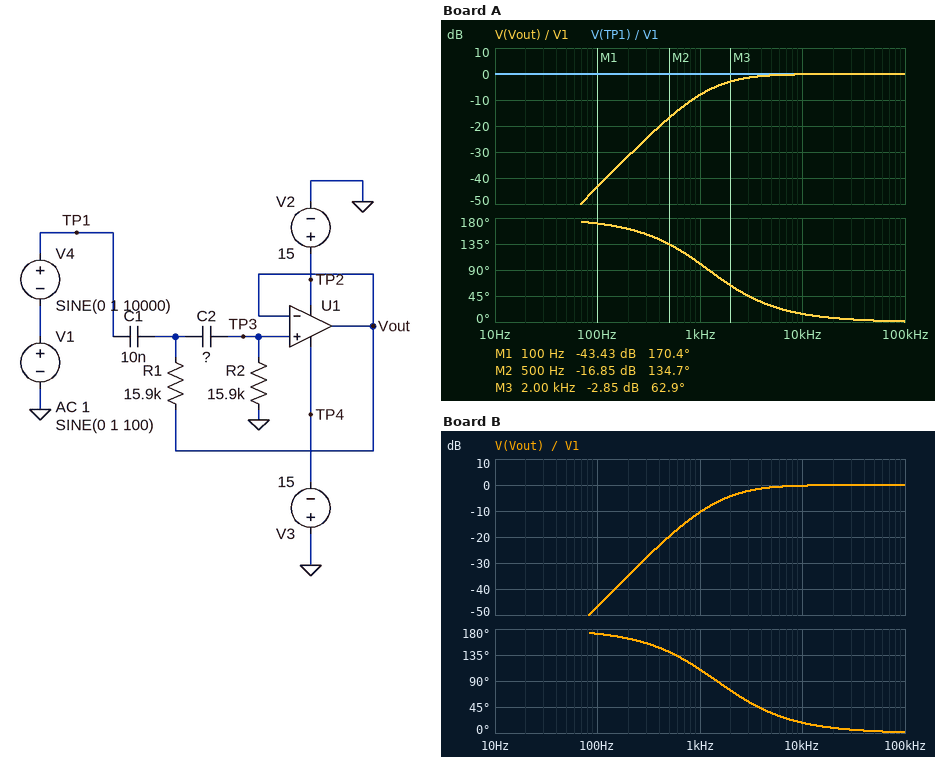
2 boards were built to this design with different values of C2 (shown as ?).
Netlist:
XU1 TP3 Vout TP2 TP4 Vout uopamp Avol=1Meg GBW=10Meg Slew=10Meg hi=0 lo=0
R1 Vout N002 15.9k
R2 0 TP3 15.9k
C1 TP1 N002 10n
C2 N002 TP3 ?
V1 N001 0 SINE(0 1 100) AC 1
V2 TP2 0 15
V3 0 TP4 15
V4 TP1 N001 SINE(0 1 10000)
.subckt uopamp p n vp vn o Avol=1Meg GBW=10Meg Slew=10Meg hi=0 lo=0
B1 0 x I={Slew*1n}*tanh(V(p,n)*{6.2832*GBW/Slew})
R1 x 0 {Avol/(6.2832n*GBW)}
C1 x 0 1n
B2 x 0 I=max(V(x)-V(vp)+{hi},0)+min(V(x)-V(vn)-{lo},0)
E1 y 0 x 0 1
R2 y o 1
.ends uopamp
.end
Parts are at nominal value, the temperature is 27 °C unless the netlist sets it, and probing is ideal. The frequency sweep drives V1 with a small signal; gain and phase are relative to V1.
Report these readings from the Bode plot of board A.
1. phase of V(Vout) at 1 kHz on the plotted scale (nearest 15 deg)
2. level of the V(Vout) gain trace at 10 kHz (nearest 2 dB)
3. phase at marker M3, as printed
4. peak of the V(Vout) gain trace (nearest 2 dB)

105 deg
0 dB
62.9 deg
0 dB
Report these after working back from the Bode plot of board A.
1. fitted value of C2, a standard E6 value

6.8 nF
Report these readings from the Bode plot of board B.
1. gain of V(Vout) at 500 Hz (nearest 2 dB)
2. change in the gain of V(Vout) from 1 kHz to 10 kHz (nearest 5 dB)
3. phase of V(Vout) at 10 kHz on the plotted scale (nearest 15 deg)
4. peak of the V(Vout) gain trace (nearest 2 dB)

-20 dB
10 dB
15 deg
0 dB
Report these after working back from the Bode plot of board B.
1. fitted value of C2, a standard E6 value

4.7 nF
